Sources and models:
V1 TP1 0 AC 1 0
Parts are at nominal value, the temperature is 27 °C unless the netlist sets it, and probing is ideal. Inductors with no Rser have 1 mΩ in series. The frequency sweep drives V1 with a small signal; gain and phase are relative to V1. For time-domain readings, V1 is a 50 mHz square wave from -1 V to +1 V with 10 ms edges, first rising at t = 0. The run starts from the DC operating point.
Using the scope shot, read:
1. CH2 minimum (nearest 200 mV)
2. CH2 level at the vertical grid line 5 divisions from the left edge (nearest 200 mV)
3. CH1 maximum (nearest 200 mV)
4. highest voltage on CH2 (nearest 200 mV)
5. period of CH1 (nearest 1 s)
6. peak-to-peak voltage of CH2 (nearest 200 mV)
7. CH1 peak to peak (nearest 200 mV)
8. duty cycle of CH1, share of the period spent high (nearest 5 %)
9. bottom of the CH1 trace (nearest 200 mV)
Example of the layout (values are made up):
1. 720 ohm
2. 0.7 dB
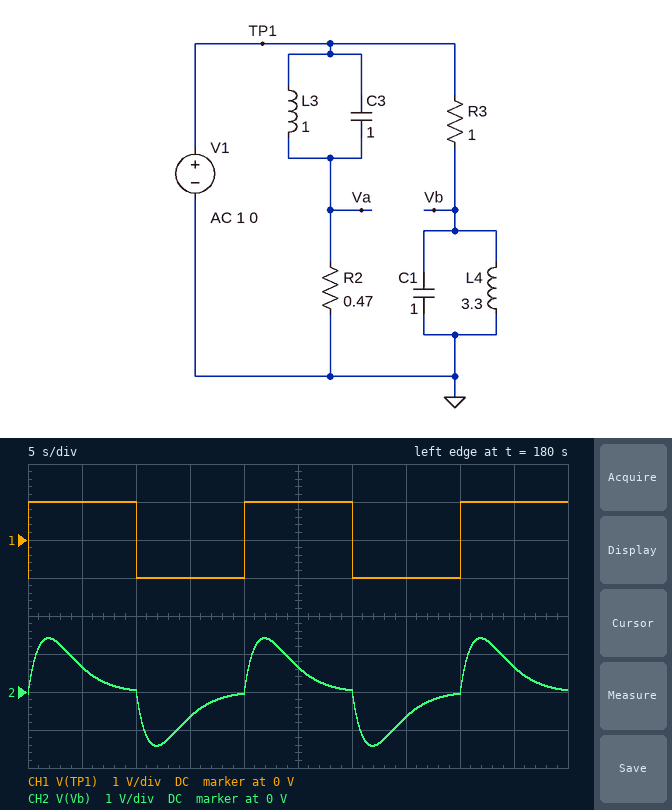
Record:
1. -1.4 V
2. 600 mV
3. 1.0 V
4. 1.4 V
5. 20 s
6. 2.8 V
7. 2.0 V
8. 50 %
9. -1.0 V
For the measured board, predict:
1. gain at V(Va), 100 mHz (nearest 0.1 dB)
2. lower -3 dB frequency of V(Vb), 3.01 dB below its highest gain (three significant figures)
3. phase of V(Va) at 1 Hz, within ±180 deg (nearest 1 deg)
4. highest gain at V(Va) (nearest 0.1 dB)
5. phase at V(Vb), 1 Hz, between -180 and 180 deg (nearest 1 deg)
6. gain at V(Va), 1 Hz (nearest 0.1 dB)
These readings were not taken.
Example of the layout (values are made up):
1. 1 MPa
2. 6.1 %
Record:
1. -7.7 dB
2. 38.8 mHz
3. 19 deg
4. 0 dB
5. -81 deg
6. -0.5 dB
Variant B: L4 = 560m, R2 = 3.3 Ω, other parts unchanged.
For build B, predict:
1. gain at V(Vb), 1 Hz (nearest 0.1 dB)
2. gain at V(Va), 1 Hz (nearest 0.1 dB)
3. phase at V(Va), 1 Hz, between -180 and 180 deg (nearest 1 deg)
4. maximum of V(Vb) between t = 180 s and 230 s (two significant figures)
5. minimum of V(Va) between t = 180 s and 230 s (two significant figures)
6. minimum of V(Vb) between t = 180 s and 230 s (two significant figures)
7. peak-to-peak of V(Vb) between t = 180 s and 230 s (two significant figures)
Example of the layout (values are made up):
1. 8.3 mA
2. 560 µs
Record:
1. -15.7 dB
2. 0 dB
3. 3 deg
4. 920 mV
5. -1.4 V
6. -920 mV
7. 1.8 V
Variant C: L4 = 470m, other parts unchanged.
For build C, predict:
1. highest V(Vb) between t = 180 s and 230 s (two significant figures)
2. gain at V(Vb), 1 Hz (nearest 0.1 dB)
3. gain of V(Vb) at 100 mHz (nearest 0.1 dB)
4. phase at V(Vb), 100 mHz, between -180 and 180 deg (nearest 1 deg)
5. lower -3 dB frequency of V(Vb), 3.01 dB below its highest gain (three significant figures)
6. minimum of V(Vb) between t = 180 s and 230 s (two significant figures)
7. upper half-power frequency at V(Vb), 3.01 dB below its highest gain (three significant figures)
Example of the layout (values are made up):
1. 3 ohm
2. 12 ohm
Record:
1. 870 mV
2. -15.6 dB
3. -9.4 dB
4. 70 deg
5. 166 mHz
6. -870 mV
7. 325 mHz
